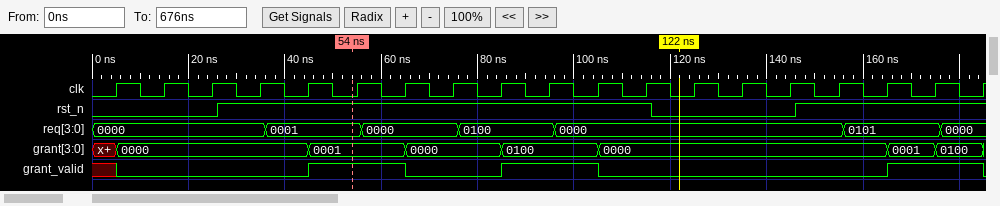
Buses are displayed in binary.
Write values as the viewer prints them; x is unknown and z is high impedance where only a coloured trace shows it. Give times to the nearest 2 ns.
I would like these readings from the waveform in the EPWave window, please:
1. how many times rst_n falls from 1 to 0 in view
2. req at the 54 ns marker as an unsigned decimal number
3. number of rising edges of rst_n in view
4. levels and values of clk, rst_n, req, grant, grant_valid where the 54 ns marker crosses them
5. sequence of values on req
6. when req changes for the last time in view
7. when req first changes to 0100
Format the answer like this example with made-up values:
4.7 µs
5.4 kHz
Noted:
1
1
2
clk=0, rst_n=1, req=0001, grant=0001, grant_valid=1
0000, 0001, 0000, 0100, 0000, 0101, 0000
176 ns
76 ns
